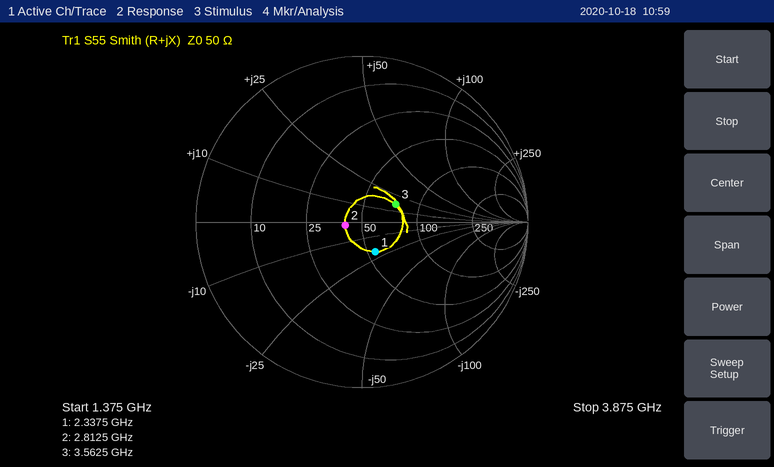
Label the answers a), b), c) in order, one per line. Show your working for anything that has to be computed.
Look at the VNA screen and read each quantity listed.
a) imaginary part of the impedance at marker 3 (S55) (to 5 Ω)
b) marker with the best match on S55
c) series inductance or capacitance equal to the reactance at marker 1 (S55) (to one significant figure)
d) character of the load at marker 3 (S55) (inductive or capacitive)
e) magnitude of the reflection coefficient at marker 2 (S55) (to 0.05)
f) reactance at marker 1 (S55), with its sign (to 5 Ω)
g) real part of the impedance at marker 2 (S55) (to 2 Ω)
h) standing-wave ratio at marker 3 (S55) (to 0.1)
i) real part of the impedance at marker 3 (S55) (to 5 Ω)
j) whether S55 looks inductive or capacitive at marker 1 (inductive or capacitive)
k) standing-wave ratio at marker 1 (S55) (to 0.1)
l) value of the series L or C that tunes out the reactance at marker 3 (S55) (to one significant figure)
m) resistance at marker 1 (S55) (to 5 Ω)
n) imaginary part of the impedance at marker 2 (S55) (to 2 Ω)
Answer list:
a) +15 Ω
b) marker 2
c) C = 1/(2π × 2.3375 GHz × 20 Ω) ≈ 3 pF
d) inductive
e) 0.10
f) -20 Ω
g) 40 Ω
h) 1.6
i) 75 Ω
j) capacitive
k) 1.5
l) C = 1/(2π × 3.5625 GHz × 15 Ω) ≈ 3 pF
m) 55 Ω
n) -2 Ω
